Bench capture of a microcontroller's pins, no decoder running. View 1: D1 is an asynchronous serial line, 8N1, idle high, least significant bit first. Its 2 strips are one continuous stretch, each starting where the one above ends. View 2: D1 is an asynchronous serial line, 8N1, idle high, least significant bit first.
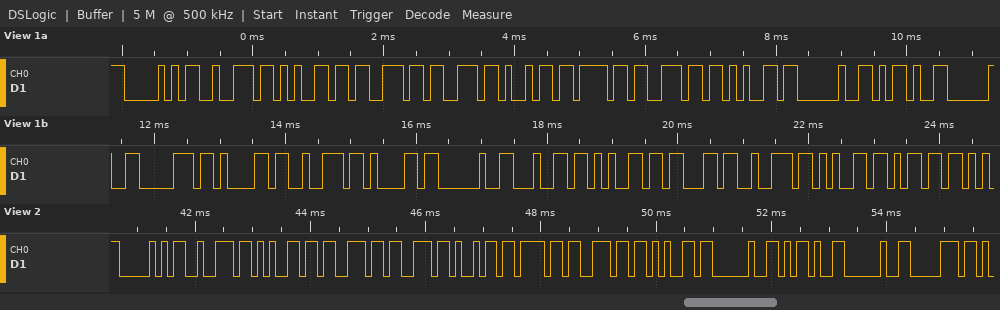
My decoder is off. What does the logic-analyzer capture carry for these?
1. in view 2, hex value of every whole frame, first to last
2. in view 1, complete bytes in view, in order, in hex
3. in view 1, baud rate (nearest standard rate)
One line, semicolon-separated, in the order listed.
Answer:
0x50 0x72 0x65 0x73 0x73 0x69 0x6F 0x6E 0x65 0x20 0x2D 0x20 0x70; 50 72 65 73 73 69 6F 6E 65 20 2D 20 70 61 72 61 20 64 65 63 72 65 6D; 9600 baud
